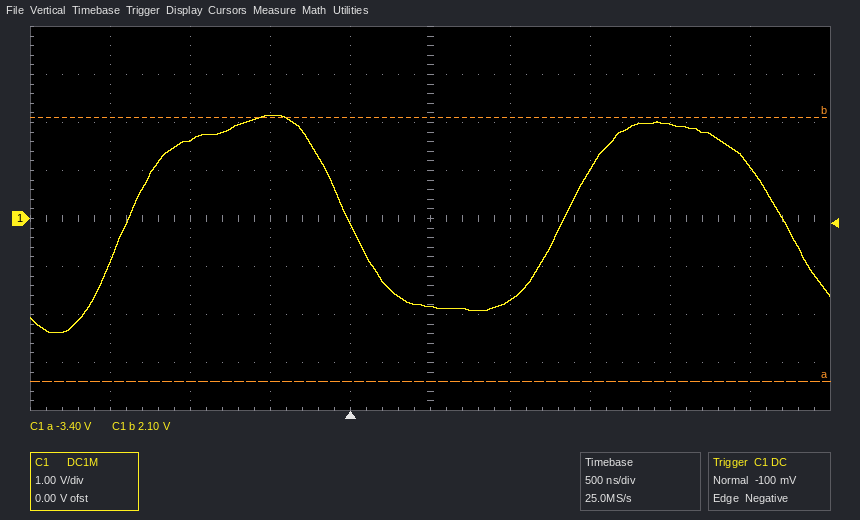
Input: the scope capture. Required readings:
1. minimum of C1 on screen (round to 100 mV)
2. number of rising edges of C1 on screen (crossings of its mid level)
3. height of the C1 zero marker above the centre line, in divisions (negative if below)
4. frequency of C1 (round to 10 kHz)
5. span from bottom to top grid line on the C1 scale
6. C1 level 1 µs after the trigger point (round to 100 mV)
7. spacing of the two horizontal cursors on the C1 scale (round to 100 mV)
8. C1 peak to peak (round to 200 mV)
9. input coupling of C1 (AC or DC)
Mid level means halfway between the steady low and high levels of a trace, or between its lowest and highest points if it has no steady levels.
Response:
-2.4 V
2
0.0 div
370 kHz
8 V
-1.7 V
5.5 V
4.6 V
DC
